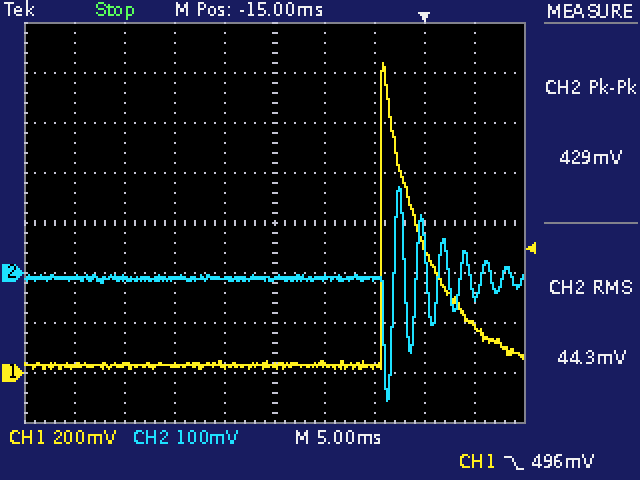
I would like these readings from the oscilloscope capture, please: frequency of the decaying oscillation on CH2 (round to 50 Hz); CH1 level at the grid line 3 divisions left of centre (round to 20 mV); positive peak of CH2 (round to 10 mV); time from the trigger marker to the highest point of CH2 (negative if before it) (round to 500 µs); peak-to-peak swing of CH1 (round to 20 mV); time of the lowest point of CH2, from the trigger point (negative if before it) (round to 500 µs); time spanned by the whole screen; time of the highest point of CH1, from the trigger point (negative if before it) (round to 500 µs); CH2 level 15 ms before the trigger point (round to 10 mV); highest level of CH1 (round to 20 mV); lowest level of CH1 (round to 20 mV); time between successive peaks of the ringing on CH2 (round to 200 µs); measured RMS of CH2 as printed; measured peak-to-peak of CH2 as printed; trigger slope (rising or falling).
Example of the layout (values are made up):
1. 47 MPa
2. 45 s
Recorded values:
1. 450 Hz
2. 40 mV
3. 170 mV
4. -2.5 ms
5. 1.22 V
6. -3.5 ms
7. 50 ms
8. -4.0 ms
9. -10 mV
10. 1.24 V
11. 20 mV
12. 2.2 ms
13. 44.3 mV
14. 429 mV
15. falling
